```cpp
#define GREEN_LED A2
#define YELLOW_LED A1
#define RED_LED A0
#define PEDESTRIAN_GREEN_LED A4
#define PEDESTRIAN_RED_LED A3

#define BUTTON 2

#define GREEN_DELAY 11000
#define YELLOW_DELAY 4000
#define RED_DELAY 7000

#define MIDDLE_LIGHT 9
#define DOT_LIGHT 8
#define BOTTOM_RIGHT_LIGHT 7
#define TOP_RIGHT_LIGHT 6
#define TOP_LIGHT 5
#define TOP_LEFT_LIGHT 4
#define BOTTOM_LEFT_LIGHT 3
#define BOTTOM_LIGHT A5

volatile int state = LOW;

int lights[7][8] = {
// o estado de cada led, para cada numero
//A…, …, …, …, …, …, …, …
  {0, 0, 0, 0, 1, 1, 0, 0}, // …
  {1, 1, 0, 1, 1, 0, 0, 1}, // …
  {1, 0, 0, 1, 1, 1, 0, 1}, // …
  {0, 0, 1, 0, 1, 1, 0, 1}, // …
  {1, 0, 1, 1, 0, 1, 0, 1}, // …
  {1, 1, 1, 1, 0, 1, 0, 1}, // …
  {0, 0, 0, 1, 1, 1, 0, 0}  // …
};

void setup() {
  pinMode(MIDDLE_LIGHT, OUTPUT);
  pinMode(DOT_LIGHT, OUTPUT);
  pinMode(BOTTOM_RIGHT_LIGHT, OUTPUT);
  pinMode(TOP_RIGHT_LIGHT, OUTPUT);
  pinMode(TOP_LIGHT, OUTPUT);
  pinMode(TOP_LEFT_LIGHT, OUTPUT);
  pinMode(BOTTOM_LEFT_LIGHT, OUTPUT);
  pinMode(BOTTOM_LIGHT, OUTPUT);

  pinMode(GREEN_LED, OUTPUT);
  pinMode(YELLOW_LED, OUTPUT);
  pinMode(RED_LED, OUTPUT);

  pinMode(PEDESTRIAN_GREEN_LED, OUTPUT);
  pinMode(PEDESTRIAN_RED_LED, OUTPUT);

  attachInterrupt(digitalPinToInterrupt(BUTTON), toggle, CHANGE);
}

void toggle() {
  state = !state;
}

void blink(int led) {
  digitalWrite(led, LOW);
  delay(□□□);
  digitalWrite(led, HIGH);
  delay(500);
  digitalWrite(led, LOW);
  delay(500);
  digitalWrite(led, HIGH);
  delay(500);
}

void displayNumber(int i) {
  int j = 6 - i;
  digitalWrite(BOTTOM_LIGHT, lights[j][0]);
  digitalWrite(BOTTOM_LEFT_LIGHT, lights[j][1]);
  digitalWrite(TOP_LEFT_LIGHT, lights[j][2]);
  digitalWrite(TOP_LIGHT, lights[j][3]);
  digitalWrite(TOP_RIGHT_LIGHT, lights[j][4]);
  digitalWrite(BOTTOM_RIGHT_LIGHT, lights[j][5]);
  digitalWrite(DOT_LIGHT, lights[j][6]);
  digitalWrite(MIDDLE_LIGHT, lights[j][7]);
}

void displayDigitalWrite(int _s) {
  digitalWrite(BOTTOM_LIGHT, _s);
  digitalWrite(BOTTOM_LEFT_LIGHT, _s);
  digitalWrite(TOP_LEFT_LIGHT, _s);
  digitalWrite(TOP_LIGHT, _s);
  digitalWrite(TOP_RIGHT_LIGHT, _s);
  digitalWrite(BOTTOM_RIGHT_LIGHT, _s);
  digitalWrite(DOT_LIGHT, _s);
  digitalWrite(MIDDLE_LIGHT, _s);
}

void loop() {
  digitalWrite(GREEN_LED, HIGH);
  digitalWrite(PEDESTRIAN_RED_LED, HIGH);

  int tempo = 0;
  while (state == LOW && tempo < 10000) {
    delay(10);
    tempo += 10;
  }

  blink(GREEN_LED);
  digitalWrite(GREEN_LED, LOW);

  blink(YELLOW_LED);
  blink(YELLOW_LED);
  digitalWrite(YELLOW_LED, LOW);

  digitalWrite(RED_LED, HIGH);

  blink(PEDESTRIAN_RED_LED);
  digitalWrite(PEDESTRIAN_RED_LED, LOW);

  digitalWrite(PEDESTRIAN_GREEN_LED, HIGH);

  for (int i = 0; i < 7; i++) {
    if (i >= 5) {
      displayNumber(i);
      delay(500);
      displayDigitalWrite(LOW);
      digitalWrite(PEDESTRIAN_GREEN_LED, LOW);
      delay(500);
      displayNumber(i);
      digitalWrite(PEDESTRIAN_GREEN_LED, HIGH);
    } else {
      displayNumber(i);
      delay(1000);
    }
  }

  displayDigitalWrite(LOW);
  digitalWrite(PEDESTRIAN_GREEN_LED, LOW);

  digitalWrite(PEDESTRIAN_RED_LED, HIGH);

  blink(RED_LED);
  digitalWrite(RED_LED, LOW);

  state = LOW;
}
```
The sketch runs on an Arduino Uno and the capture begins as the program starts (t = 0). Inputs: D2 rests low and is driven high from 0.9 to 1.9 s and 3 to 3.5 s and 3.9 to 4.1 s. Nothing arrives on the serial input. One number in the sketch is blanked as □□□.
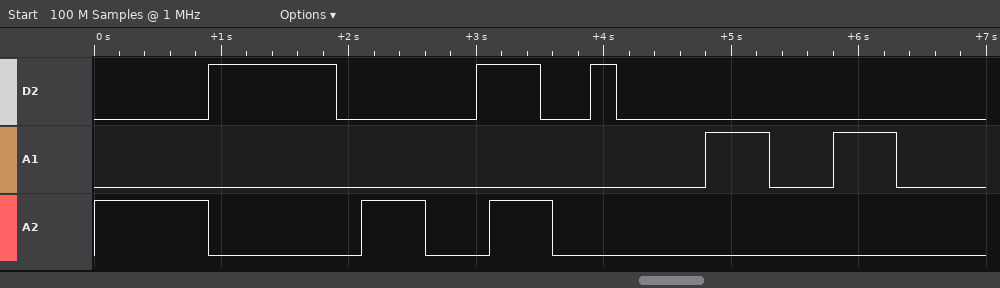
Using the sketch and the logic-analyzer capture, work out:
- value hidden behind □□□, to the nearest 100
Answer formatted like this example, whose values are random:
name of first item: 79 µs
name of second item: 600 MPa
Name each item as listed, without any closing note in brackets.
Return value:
value hidden behind □□□, to the nearest 100: 1200
